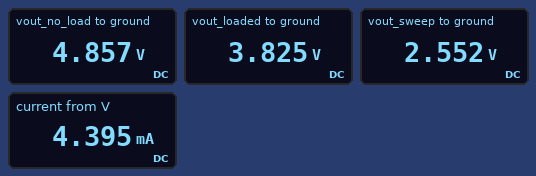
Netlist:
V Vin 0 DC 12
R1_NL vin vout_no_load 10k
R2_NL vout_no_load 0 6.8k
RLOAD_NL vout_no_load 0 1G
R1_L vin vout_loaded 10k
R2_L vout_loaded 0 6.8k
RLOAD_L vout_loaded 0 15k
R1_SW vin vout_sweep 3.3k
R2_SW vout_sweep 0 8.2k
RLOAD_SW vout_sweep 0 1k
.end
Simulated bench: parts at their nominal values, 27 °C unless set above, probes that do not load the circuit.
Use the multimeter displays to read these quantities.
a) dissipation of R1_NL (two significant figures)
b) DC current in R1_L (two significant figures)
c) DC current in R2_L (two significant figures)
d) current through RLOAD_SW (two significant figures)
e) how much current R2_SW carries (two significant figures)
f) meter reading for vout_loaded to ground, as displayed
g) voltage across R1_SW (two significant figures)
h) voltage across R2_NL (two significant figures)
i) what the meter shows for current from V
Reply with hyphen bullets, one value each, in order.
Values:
- 5.1 mW
- 820 µA
- 560 µA
- 2.6 mA
- 310 µA
- 3.825 V
- 9.4 V
- 4.9 V
- 4.395 mA
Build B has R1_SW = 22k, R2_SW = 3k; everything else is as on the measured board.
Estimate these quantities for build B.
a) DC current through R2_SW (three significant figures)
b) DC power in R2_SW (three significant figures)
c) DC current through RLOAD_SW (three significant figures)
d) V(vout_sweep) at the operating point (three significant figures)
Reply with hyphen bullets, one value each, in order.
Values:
- 132 µA
- 52.2 µW
- 396 µA
- 396 mV
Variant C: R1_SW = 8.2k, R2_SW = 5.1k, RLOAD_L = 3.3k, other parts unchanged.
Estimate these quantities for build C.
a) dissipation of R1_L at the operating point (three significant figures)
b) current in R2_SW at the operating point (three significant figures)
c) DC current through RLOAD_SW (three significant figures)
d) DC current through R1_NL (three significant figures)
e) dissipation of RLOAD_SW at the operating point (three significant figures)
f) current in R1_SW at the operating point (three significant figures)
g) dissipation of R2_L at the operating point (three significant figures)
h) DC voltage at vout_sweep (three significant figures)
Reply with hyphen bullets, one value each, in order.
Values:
- 9.64 mW
- 218 µA
- 1.11 mA
- 714 µA
- 1.23 mW
- 1.33 mA
- 700 µW
- 1.11 V
